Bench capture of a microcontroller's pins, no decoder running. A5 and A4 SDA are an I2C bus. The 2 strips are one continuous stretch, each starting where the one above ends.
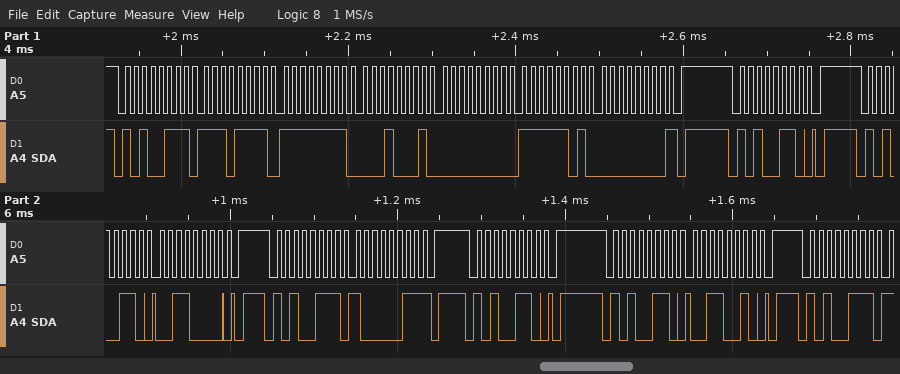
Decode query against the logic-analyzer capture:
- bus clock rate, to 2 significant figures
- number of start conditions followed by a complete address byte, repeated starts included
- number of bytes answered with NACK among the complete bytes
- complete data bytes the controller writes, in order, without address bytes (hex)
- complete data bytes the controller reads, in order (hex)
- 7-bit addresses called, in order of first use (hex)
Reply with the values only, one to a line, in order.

100 kHz
7
2
30 32
EF FF 11 00 FD 00 83
0x53
